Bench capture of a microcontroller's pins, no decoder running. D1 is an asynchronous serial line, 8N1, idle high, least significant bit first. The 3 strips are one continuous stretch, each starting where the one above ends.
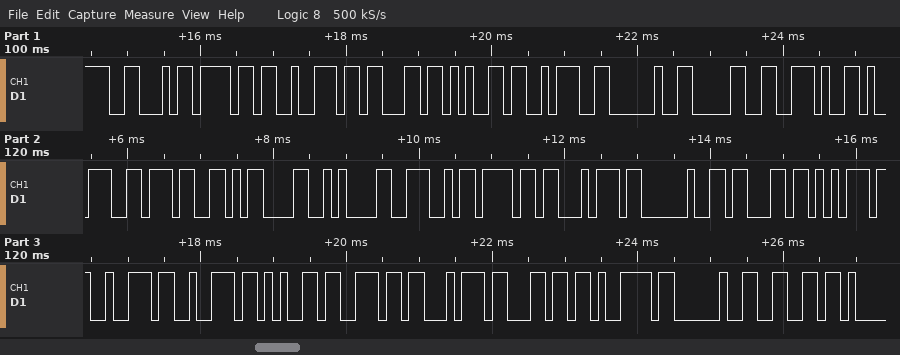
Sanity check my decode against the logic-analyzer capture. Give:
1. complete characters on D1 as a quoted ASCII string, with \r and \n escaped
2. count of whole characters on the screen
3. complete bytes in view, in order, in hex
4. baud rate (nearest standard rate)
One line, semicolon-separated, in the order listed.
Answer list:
"Force: 0.97\r\nNot currently f"; 28; 46 6F 72 63 65 3A 20 30 2E 39 37 0D 0A 4E 6F 74 20 63 75 72 72 65 6E 74 6C 79 20 66; 9600 baud
